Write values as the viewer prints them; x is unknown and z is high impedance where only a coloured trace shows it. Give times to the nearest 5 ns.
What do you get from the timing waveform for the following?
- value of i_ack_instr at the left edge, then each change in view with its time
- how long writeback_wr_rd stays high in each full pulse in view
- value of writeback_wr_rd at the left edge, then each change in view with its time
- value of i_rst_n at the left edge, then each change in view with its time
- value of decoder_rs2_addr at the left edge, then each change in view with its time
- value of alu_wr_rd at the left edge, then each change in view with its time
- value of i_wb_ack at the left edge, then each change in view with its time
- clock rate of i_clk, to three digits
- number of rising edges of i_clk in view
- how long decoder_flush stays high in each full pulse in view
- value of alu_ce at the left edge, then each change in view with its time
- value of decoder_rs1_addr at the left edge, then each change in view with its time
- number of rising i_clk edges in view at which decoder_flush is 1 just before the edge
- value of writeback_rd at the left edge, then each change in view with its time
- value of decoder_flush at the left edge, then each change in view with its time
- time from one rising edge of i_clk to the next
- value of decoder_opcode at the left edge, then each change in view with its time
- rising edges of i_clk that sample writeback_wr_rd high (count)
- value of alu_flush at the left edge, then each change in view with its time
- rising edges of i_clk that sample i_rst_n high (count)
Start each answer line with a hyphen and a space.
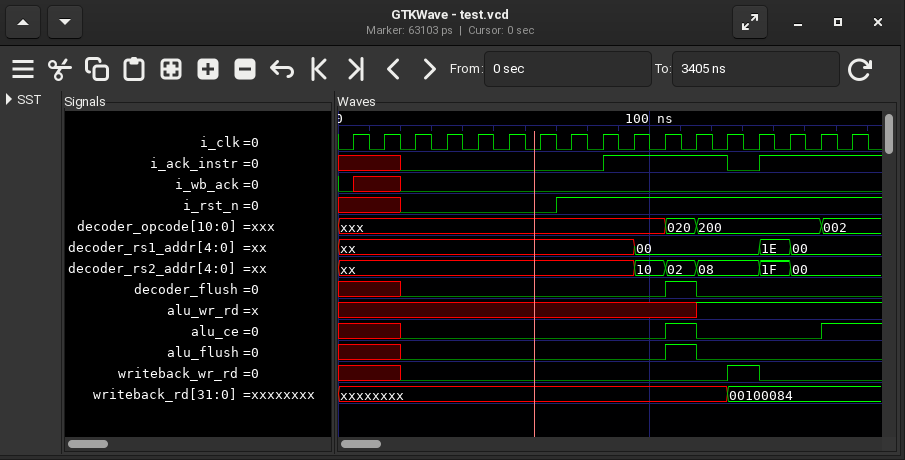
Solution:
- x, 0 at 20 ns, 1 at 85 ns, 0 at 125 ns, 1 at 135 ns
- 10 ns
- x, 0 at 20 ns, 1 at 125 ns, 0 at 135 ns
- x, 0 at 20 ns, 1 at 70 ns
- xx, 10 at 95 ns, 02 at 105 ns, 08 at 115 ns, 1F at 135 ns, 00 at 145 ns
- x, 1 at 115 ns
- 0, x at 5 ns, 0 at 20 ns
- 100 MHz
- 17
- 10 ns
- x, 0 at 20 ns, 1 at 105 ns, 0 at 115 ns, 1 at 155 ns
- xx, 00 at 95 ns, 1E at 135 ns, 00 at 145 ns
- 1
- xxxxxxxx, 00100084 at 125 ns
- x, 0 at 20 ns, 1 at 105 ns, 0 at 115 ns
- 10 ns
- xxx, 020 at 105 ns, 200 at 115 ns, 002 at 155 ns
- 1
- x, 0 at 20 ns, 1 at 105 ns, 0 at 115 ns
- 10
